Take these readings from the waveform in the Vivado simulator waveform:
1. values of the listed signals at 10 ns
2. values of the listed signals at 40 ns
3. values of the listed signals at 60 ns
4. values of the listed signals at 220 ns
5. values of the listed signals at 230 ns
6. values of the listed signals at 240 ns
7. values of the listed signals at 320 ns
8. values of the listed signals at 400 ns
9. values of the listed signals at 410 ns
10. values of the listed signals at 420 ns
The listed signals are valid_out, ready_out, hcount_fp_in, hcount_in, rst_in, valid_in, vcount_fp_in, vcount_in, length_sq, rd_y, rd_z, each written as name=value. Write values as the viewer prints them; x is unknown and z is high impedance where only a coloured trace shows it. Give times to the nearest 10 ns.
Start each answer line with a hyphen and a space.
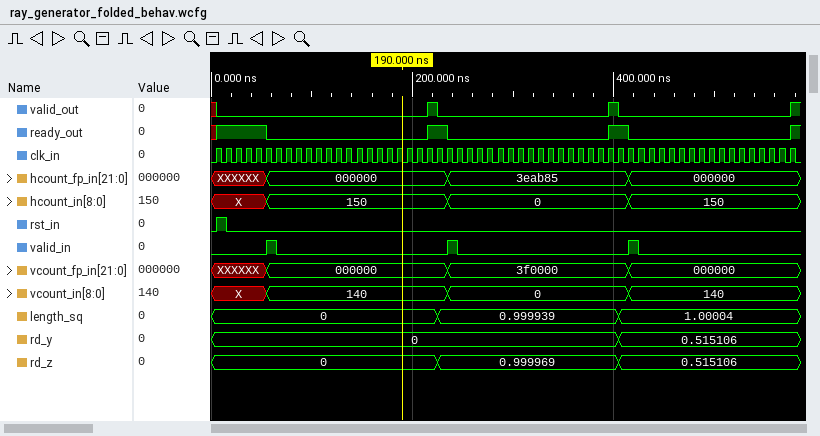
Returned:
- valid_out=0, ready_out=1, hcount_fp_in=XXXXXX, hcount_in=X, rst_in=1, valid_in=0, vcount_fp_in=XXXXXX, vcount_in=X, length_sq=0, rd_y=0, rd_z=0
- valid_out=0, ready_out=1, hcount_fp_in=XXXXXX, hcount_in=X, rst_in=0, valid_in=0, vcount_fp_in=XXXXXX, vcount_in=X, length_sq=0, rd_y=0, rd_z=0
- valid_out=0, ready_out=0, hcount_fp_in=000000, hcount_in=150, rst_in=0, valid_in=1, vcount_fp_in=000000, vcount_in=140, length_sq=0, rd_y=0, rd_z=0
- valid_out=1, ready_out=1, hcount_fp_in=000000, hcount_in=150, rst_in=0, valid_in=0, vcount_fp_in=000000, vcount_in=140, length_sq=0, rd_y=0, rd_z=0
- valid_out=0, ready_out=1, hcount_fp_in=000000, hcount_in=150, rst_in=0, valid_in=0, vcount_fp_in=000000, vcount_in=140, length_sq=0.999939, rd_y=0, rd_z=0.999969
- valid_out=0, ready_out=0, hcount_fp_in=3eab85, hcount_in=0, rst_in=0, valid_in=1, vcount_fp_in=3f0000, vcount_in=0, length_sq=0.999939, rd_y=0, rd_z=0.999969
- valid_out=0, ready_out=0, hcount_fp_in=3eab85, hcount_in=0, rst_in=0, valid_in=0, vcount_fp_in=3f0000, vcount_in=0, length_sq=0.999939, rd_y=0, rd_z=0.999969
- valid_out=1, ready_out=1, hcount_fp_in=3eab85, hcount_in=0, rst_in=0, valid_in=0, vcount_fp_in=3f0000, vcount_in=0, length_sq=0.999939, rd_y=0, rd_z=0.999969
- valid_out=0, ready_out=1, hcount_fp_in=3eab85, hcount_in=0, rst_in=0, valid_in=0, vcount_fp_in=3f0000, vcount_in=0, length_sq=1.00004, rd_y=0.515106, rd_z=0.515106
- valid_out=0, ready_out=0, hcount_fp_in=000000, hcount_in=150, rst_in=0, valid_in=1, vcount_fp_in=000000, vcount_in=140, length_sq=1.00004, rd_y=0.515106, rd_z=0.515106
